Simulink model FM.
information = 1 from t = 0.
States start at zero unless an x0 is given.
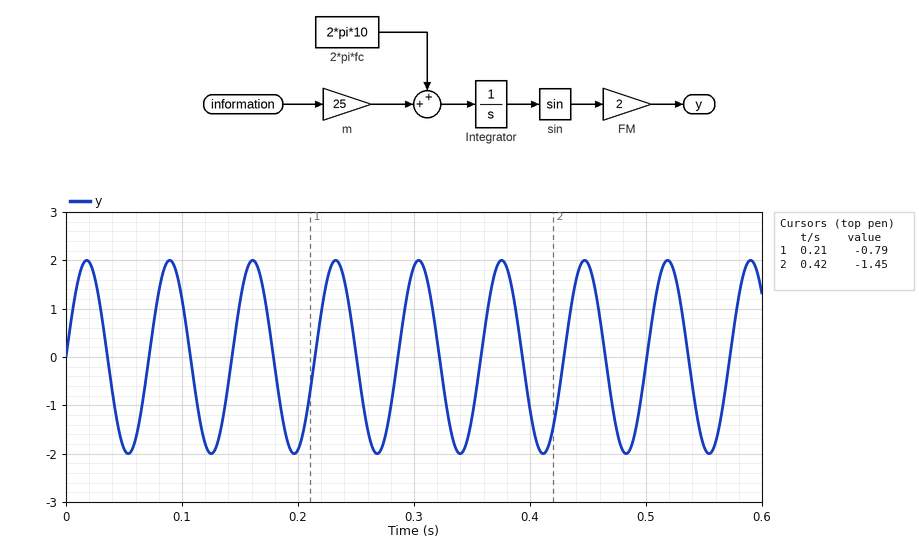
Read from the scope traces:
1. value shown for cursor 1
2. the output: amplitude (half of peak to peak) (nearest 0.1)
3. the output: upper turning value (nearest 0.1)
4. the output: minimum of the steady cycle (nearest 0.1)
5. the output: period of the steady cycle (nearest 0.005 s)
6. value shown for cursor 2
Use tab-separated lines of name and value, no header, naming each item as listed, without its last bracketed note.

value shown for cursor 1	-0.79
the output: amplitude (half of peak to peak)	2.0
the output: upper turning value	2.0
the output: minimum of the steady cycle	-2.0
the output: period of the steady cycle	0.070 s
value shown for cursor 2	-1.45
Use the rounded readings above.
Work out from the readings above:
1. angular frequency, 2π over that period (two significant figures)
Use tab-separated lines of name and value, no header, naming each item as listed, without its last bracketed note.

angular frequency, 2π over that period	90 rad/s
